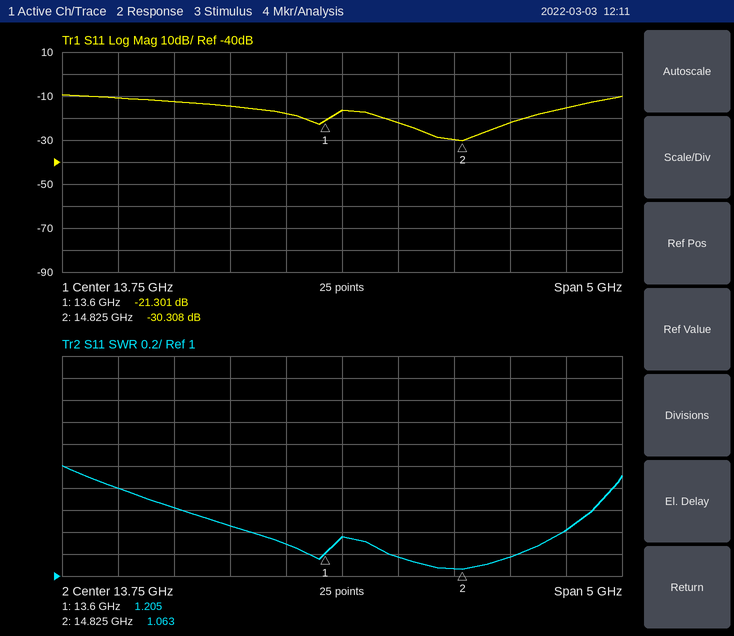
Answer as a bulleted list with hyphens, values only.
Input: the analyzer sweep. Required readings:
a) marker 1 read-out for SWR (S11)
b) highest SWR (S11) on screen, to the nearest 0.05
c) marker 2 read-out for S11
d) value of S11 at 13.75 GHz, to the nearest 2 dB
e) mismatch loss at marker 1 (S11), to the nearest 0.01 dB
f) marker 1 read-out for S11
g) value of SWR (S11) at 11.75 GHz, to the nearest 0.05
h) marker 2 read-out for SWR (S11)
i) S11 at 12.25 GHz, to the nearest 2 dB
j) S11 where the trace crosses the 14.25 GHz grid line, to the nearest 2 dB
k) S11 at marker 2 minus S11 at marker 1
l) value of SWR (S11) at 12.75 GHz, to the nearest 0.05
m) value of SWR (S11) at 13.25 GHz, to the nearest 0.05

- 1.205
- 2.00
- -30.308 dB
- -16 dB
- 0.03 dB
- -21.301 dB
- 1.80
- 1.063
- -12 dB
- -22 dB
- -9.007 dB
- 1.45
- 1.30
